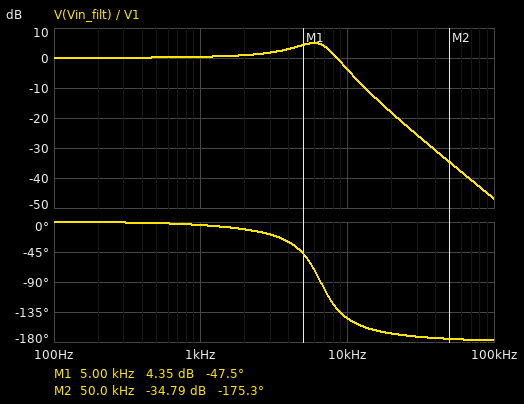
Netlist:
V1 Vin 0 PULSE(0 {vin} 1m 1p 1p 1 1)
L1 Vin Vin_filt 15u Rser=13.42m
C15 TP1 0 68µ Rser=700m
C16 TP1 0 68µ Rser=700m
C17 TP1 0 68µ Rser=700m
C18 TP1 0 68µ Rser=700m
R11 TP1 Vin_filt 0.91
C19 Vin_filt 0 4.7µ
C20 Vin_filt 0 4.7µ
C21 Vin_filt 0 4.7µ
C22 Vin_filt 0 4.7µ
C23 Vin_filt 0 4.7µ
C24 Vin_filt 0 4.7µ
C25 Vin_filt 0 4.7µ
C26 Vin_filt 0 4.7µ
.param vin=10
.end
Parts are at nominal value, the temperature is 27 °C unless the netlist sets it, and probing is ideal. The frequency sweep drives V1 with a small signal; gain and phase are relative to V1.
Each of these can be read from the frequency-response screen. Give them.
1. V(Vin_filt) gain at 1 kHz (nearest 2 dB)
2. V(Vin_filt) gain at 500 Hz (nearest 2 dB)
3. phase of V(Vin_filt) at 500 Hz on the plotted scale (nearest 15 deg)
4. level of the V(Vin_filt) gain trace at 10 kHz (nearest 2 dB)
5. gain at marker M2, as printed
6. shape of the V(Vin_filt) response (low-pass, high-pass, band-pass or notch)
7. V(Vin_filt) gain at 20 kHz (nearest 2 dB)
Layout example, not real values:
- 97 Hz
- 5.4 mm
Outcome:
- 0 dB
- 0 dB
- 0 deg
- -4 dB
- -34.79 dB
- low-pass
- -18 dB
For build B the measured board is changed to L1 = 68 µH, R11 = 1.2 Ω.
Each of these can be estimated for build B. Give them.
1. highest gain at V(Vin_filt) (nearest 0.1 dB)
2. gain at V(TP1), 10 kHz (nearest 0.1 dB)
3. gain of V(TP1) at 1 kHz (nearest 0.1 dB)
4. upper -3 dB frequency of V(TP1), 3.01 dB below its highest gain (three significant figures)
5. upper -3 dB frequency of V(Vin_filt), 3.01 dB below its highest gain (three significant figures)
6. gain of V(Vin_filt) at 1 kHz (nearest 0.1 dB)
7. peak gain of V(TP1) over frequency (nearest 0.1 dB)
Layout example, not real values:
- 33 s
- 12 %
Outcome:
- 2.3 dB
- -37.2 dB
- -6.3 dB
- 521 Hz
- 3.40 kHz
- 1.5 dB
- 0 dB
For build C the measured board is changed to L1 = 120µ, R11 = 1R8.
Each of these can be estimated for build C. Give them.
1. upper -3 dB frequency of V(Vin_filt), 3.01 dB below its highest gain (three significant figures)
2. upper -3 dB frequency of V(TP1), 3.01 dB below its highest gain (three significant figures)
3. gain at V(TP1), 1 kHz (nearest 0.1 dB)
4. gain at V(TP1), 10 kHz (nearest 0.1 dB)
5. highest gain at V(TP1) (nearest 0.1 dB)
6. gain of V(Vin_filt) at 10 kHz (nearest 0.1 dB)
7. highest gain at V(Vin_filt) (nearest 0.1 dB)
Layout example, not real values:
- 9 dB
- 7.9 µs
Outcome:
- 2.62 kHz
- 349 Hz
- -8.7 dB
- -45.4 dB
- 0 dB
- -24.8 dB
- 2.6 dB
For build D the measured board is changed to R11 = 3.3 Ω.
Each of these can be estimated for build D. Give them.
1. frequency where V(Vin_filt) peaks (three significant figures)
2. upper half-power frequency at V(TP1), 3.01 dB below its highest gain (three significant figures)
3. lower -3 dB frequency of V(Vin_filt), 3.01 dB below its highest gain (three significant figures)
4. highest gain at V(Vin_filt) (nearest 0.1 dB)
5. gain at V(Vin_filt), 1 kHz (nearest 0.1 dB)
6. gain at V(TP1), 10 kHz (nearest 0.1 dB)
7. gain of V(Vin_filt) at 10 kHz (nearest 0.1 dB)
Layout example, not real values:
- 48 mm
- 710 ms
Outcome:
- 6.63 kHz
- 169 Hz
- 5.91 kHz
- 13.9 dB
- 0.2 dB
- -27.5 dB
- -2.0 dB
